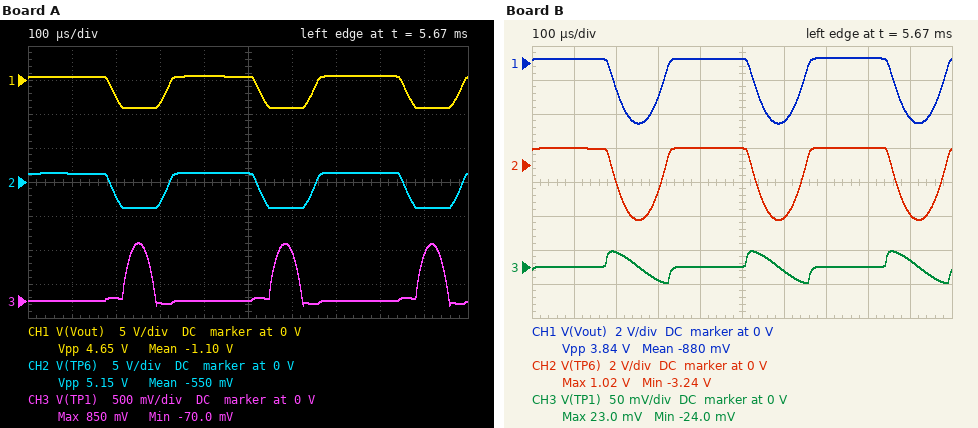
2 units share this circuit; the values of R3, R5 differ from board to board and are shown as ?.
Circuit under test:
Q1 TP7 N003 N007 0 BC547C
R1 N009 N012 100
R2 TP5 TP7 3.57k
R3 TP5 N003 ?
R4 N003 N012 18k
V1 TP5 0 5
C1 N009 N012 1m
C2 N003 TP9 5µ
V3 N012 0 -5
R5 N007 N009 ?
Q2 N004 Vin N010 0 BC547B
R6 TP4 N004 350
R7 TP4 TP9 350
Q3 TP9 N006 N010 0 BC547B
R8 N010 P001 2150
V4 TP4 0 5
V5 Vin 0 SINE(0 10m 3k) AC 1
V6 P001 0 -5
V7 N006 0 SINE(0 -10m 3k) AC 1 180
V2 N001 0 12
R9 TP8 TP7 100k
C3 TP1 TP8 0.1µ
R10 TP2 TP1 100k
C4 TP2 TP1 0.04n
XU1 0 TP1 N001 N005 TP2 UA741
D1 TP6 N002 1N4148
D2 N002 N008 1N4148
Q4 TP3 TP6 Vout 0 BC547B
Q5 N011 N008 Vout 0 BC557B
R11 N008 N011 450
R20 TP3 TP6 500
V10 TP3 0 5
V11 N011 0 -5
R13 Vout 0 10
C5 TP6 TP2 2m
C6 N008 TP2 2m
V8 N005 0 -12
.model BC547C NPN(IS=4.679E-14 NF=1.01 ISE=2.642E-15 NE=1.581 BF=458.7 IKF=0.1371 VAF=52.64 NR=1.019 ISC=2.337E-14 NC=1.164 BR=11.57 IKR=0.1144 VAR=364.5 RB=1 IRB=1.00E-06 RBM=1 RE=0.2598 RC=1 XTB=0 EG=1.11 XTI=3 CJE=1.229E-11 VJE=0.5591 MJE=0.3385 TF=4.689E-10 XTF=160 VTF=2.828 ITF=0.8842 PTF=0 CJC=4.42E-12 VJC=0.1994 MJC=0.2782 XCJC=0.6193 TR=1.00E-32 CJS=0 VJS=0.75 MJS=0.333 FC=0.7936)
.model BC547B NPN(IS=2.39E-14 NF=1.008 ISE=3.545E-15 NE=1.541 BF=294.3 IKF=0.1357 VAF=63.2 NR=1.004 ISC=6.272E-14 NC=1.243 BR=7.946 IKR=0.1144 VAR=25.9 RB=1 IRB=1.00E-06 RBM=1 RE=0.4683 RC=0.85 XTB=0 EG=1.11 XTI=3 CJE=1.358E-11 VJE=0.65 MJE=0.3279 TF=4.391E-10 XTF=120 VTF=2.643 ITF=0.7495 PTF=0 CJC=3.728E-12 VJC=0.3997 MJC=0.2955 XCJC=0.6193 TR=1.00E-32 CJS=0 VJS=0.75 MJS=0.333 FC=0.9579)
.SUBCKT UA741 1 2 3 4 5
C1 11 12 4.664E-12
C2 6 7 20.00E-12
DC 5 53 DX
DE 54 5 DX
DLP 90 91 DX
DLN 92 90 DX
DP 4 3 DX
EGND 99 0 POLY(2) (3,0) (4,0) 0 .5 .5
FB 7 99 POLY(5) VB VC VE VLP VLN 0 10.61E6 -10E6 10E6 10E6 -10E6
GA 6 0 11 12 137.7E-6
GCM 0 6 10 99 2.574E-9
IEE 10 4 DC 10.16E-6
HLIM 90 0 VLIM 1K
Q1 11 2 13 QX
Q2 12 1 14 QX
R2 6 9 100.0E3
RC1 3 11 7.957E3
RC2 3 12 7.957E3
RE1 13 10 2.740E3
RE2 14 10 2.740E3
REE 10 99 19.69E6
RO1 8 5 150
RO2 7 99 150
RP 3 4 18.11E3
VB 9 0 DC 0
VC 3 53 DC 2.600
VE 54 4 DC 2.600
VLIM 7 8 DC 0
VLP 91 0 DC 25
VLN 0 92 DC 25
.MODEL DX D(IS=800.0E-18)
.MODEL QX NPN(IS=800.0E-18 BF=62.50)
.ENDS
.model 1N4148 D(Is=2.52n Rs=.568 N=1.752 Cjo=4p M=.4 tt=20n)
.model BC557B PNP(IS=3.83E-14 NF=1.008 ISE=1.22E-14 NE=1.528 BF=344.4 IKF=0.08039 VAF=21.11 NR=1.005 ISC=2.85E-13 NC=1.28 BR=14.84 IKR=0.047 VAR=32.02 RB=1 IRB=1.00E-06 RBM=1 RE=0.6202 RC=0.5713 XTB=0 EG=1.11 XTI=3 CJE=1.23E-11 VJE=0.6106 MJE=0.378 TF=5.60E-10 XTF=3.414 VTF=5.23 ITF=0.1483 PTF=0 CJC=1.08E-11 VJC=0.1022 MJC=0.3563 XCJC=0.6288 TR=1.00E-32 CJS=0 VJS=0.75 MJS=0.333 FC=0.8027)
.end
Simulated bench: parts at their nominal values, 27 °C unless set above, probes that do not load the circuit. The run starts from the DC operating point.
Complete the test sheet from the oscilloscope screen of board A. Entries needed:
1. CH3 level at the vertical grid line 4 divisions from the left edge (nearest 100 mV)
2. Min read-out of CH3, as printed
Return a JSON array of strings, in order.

["0 V", "-70.0 mV"]
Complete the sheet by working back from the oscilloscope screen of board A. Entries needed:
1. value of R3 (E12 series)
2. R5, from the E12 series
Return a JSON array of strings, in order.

["56 kΩ", "33 Ω"]
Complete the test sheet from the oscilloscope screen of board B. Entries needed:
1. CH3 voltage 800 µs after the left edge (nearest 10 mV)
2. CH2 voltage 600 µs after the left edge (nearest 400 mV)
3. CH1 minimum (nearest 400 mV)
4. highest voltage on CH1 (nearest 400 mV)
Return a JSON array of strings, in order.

["0 V", "-3.2 V", "-3.6 V", "400 mV"]
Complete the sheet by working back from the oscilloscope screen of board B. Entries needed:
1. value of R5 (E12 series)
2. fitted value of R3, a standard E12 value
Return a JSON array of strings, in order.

["68 Ω", "56 kΩ"]
